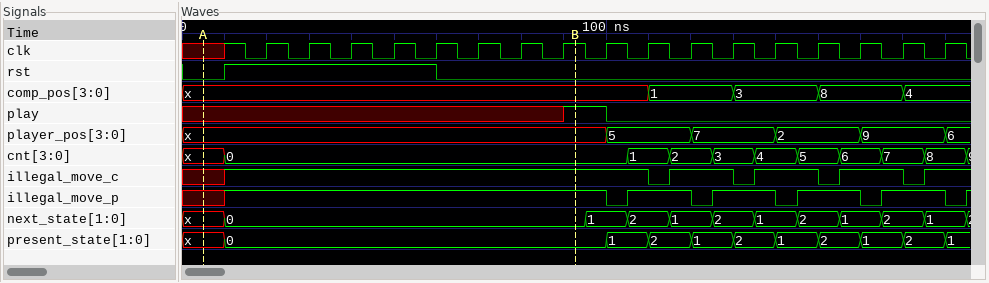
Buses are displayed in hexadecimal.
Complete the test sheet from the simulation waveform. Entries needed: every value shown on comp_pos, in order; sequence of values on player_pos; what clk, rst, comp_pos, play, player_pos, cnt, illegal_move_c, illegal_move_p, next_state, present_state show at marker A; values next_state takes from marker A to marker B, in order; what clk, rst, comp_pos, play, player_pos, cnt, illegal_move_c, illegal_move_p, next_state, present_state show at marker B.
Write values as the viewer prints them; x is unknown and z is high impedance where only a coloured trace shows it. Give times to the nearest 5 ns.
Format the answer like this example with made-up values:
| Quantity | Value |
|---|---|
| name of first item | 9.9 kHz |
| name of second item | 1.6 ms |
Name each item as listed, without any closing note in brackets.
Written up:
| Quantity | Value |
|---|---|
| every value shown on comp_pos, in order | x, 1, 3, 8, 4 |
| sequence of values on player_pos | x, 5, 7, 2, 9, 6 |
| what clk, rst, comp_pos, play, player_pos, cnt, illegal_move_c, illegal_move_p, next_state, present_state show at marker A | clk=x, rst=0, comp_pos=x, play=x, player_pos=x, cnt=x, illegal_move_c=x, illegal_move_p=x, next_state=x, present_state=x |
| values next_state takes from marker A to marker B, in order | x, 0 |
| what clk, rst, comp_pos, play, player_pos, cnt, illegal_move_c, illegal_move_p, next_state, present_state show at marker B | clk=1, rst=0, comp_pos=x, play=1, player_pos=x, cnt=0, illegal_move_c=1, illegal_move_p=1, next_state=0, present_state=0 |
